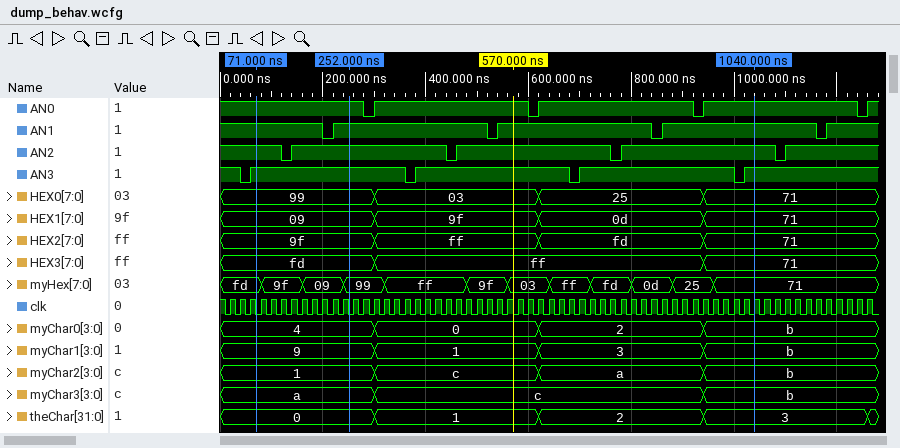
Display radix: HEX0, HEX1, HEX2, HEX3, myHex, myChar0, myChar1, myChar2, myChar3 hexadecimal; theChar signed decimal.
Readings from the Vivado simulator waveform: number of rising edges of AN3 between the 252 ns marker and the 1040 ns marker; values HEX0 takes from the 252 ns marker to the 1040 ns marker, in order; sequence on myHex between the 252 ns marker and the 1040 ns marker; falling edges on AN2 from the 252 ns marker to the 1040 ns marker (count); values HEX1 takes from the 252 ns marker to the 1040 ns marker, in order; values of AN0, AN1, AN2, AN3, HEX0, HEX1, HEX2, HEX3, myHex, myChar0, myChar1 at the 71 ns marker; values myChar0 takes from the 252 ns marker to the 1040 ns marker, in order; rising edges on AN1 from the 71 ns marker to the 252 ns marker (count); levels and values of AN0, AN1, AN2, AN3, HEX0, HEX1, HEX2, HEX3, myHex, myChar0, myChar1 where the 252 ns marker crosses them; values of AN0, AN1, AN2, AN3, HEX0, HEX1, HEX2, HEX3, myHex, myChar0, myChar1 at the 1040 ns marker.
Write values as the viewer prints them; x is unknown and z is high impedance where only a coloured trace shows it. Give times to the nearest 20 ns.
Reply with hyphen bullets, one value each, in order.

- 3
- 99, 03, 25, 71
- 99, ff, 9f, 03, ff, fd, 0d, 25, 71
- 2
- 09, 9f, 0d, 71
- AN0=1, AN1=1, AN2=1, AN3=1, HEX0=99, HEX1=09, HEX2=9f, HEX3=fd, myHex=fd, myChar0=4, myChar1=9
- 4, 0, 2, b
- 1
- AN0=1, AN1=1, AN2=1, AN3=1, HEX0=99, HEX1=09, HEX2=9f, HEX3=fd, myHex=99, myChar0=4, myChar1=9
- AN0=1, AN1=1, AN2=1, AN3=1, HEX0=71, HEX1=71, HEX2=71, HEX3=71, myHex=71, myChar0=b, myChar1=b
